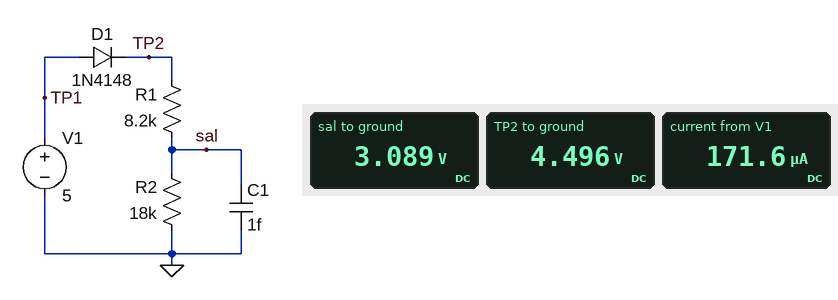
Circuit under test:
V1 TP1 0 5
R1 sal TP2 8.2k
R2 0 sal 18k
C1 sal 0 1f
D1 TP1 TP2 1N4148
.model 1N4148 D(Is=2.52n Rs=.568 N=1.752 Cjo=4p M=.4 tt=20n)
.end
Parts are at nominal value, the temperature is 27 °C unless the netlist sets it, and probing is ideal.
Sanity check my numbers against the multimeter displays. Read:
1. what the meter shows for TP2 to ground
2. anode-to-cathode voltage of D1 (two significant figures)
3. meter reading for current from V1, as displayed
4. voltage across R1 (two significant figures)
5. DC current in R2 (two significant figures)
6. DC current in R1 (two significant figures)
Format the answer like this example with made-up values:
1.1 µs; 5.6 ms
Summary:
4.496 V; 500 mV; 171.6 µA; 1.4 V; 170 µA; 170 µA
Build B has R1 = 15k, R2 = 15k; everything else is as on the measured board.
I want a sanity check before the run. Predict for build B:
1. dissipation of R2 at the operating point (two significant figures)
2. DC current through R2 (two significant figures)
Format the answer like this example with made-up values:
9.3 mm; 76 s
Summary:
340 µW; 150 µA
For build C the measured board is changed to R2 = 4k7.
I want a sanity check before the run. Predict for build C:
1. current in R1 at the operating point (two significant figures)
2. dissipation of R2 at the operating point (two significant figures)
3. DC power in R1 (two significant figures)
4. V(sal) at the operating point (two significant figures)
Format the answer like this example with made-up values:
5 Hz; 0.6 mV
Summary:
350 µA; 560 µW; 980 µW; 1.6 V
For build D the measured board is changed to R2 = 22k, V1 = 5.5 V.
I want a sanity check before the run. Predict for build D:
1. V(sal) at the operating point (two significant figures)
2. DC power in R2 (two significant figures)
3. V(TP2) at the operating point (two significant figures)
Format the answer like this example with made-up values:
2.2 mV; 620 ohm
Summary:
3.6 V; 600 µW; 5.0 V
